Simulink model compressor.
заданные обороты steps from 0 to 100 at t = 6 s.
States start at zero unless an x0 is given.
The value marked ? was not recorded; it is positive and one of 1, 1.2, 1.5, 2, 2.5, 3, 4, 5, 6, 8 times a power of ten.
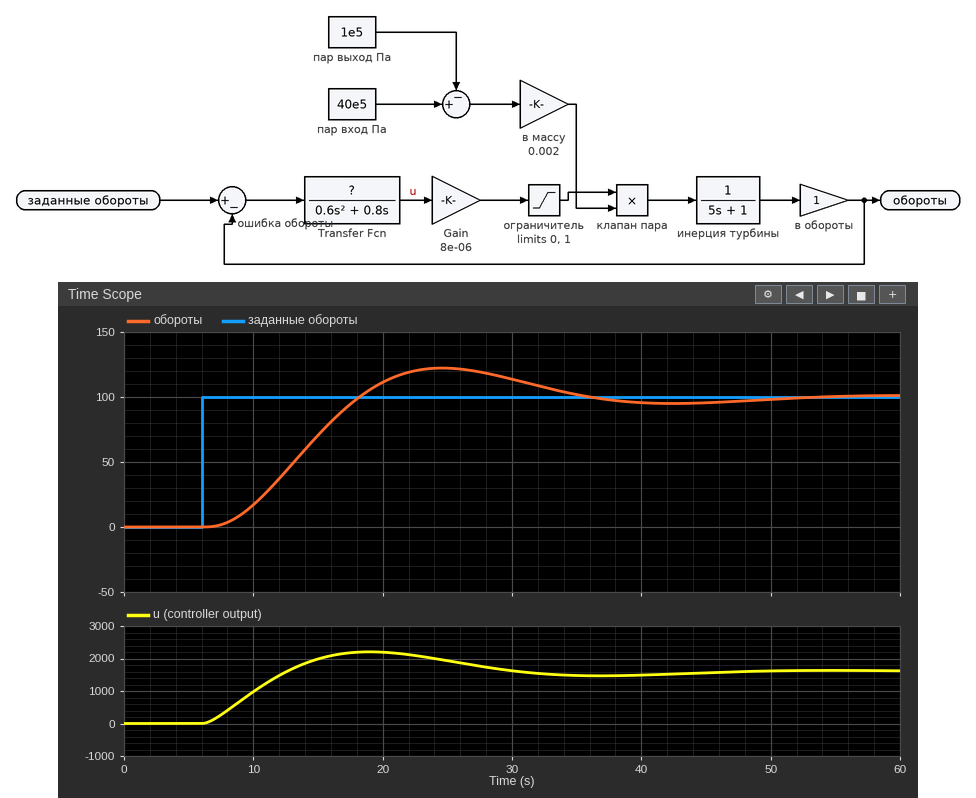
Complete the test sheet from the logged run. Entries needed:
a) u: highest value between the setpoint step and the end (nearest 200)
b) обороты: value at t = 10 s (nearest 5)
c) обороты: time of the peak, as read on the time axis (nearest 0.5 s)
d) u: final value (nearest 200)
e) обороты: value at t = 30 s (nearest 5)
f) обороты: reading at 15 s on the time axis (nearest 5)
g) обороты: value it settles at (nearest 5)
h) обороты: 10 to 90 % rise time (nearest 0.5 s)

2200
15
24.5 s
1600
115
70
100
8.0 s
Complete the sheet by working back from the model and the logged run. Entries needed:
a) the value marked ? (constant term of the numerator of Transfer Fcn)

2.5
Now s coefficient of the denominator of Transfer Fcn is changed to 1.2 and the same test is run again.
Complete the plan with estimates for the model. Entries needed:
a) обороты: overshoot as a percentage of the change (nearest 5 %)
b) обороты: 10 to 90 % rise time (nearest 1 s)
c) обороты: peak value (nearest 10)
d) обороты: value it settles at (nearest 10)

10 %
11 s
110
100
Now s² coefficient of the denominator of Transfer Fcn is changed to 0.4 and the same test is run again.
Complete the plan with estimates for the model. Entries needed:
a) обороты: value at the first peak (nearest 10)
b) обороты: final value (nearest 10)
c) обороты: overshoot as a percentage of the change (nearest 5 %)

120
100
20 %
